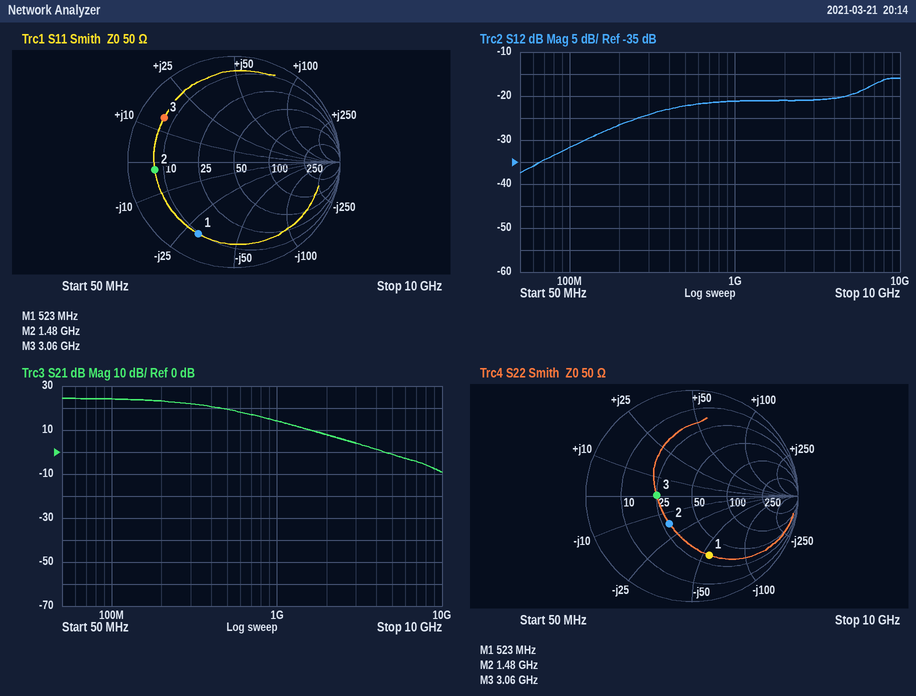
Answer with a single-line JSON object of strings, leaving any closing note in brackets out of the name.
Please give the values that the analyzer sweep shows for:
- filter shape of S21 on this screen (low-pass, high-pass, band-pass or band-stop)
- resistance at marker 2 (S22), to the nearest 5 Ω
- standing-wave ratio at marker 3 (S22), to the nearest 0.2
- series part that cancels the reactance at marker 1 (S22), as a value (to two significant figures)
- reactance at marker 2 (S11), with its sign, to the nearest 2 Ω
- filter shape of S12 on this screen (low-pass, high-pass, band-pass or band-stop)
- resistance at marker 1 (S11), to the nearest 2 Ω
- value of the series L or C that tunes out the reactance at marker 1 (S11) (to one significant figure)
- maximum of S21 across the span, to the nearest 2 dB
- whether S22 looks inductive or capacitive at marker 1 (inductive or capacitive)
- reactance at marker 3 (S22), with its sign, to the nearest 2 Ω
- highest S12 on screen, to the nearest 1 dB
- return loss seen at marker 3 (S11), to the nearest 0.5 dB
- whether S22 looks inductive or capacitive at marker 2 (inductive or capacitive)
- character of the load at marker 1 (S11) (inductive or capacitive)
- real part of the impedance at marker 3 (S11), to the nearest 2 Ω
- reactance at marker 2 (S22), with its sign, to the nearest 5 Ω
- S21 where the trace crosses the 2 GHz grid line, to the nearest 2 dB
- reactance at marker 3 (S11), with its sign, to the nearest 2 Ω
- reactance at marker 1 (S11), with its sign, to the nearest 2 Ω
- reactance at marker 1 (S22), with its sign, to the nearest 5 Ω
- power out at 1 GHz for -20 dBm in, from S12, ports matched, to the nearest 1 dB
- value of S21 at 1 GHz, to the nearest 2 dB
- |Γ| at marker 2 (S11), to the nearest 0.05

{"filter shape of S21 on this screen": "low-pass", "resistance at marker 2 (S22), to the nearest 5 Ω": "30 Ω", "standing-wave ratio at marker 3 (S22), to the nearest 0.2": "2.0", "series part that cancels the reactance at marker 1 (S22), as a value": "17 nH", "reactance at marker 2 (S11), with its sign, to the nearest 2 Ω": "-2 Ω", "filter shape of S12 on this screen": "high-pass", "resistance at marker 1 (S11), to the nearest 2 Ω": "10 Ω", "value of the series L or C that tunes out the reactance at marker 1 (S11)": "9 nH", "maximum of S21 across the span, to the nearest 2 dB": "24 dB", "whether S22 looks inductive or capacitive at marker 1": "capacitive", "reactance at marker 3 (S22), with its sign, to the nearest 2 Ω": "0 Ω", "highest S12 on screen, to the nearest 1 dB": "-16 dB", "return loss seen at marker 3 (S11), to the nearest 0.5 dB": "2.0 dB", "whether S22 looks inductive or capacitive at marker 2": "capacitive", "character of the load at marker 1 (S11)": "capacitive", "real part of the impedance at marker 3 (S11), to the nearest 2 Ω": "6 Ω", "reactance at marker 2 (S22), with its sign, to the nearest 5 Ω": "-15 Ω", "S21 where the trace crosses the 2 GHz grid line, to the nearest 2 dB": "8 dB", "reactance at marker 3 (S11), with its sign, to the nearest 2 Ω": "+14 Ω", "reactance at marker 1 (S11), with its sign, to the nearest 2 Ω": "-30 Ω", "reactance at marker 1 (S22), with its sign, to the nearest 5 Ω": "-55 Ω", "power out at 1 GHz for -20 dBm in, from S12, ports matched, to the nearest 1 dB": "-41 dBm", "value of S21 at 1 GHz, to the nearest 2 dB": "14 dB", "|Γ| at marker 2 (S11), to the nearest 0.05": "0.75"}
